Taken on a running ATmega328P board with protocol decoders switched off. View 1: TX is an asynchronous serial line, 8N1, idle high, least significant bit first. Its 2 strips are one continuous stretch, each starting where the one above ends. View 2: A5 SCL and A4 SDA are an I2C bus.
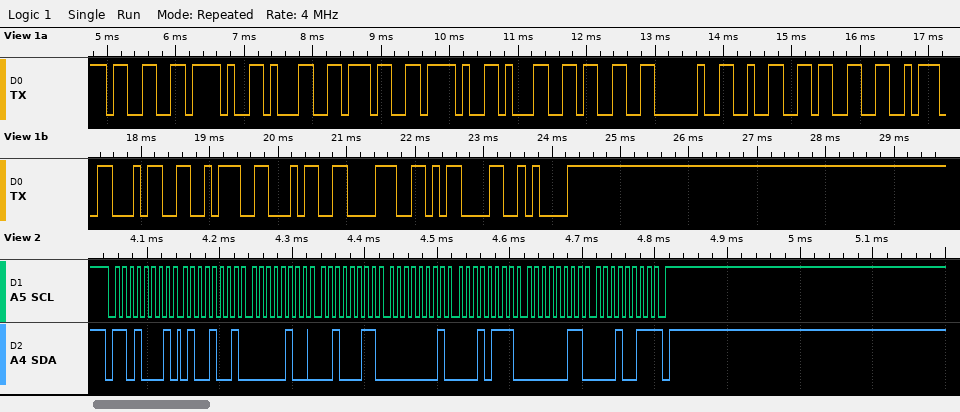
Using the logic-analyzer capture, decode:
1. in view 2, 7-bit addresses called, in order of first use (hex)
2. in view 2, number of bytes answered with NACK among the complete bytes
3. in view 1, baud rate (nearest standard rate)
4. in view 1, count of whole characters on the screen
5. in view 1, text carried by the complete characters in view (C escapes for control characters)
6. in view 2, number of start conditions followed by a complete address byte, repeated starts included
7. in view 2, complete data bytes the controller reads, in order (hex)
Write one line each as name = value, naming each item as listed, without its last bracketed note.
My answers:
in view 2, 7-bit addresses called, in order of first use = 0x68
in view 2, number of bytes answered with NACK among the complete bytes = 1
in view 1, baud rate = 9600 baud
in view 1, count of whole characters on the screen = 17
in view 1, text carried by the complete characters in view = "3/17/13 23:4:48\r\n"
in view 2, number of start conditions followed by a complete address byte, repeated starts included = 1
in view 2, complete data bytes the controller reads, in order = 49 04 23 01 17 03 13
